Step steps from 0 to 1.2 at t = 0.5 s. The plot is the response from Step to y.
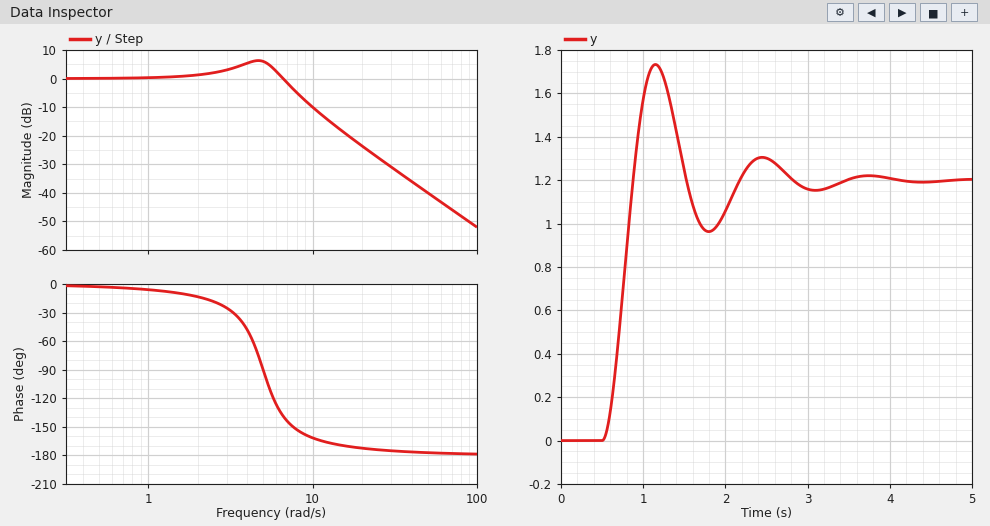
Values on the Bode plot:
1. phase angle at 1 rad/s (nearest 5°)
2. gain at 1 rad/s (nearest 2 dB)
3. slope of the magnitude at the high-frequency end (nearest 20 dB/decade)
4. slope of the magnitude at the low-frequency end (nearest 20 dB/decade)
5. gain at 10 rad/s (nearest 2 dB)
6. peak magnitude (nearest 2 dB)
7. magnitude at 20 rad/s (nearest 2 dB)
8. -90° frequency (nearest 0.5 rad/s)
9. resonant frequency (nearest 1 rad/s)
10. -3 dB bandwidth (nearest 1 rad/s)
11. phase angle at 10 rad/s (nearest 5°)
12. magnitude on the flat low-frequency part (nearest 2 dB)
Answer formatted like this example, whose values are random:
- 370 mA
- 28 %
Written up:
- -5°
- 0 dB
- -40 dB/decade
- 0 dB/decade
- -10 dB
- 6 dB
- -24 dB
- 5.0 rad/s
- 5 rad/s
- 7 rad/s
- -160°
- 0 dB
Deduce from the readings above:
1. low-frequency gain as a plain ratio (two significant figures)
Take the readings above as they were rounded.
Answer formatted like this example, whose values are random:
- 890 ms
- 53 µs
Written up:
- 1.0
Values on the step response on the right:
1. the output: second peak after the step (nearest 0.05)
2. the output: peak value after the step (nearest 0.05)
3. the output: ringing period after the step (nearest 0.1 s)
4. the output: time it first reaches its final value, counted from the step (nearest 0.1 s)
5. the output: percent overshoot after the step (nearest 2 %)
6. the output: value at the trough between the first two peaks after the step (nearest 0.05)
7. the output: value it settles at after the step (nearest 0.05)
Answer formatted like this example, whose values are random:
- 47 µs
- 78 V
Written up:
- 1.30
- 1.75
- 1.3 s
- 0.4 s
- 44 %
- 0.95
- 1.20
